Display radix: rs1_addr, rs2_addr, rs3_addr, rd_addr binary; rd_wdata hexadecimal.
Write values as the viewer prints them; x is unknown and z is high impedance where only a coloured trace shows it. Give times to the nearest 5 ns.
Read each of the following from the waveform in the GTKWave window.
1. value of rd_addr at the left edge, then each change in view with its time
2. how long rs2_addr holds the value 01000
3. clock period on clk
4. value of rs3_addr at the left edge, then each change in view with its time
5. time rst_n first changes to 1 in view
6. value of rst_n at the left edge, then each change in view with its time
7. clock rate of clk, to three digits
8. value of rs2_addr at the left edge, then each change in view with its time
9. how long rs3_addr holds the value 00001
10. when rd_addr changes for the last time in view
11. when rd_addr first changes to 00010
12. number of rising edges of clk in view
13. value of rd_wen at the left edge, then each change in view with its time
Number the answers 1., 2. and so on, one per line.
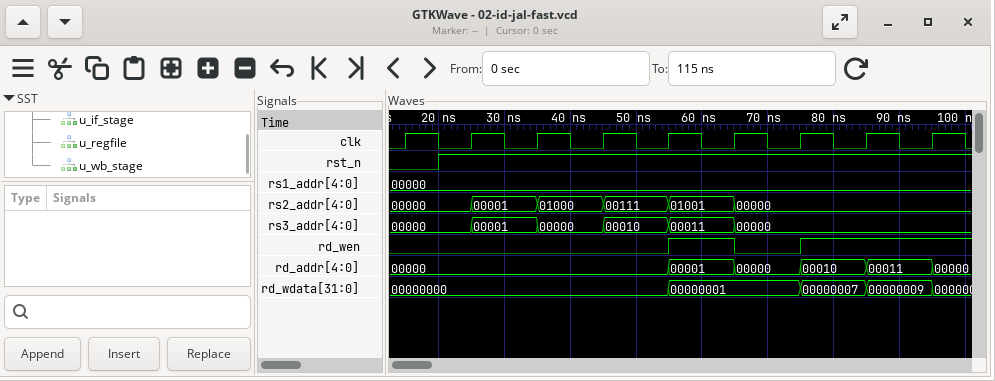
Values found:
1. 00000, 00001 at 55 ns, 00000 at 65 ns, 00010 at 75 ns, 00011 at 85 ns, 00000 at 95 ns
2. 10 ns
3. 10 ns
4. 00000, 00001 at 25 ns, 00000 at 35 ns, 00010 at 45 ns, 00011 at 55 ns, 00000 at 65 ns
5. 20 ns
6. 0, 1 at 20 ns
7. 100 MHz
8. 00000, 00001 at 25 ns, 01000 at 35 ns, 00111 at 45 ns, 01001 at 55 ns, 00000 at 65 ns
9. 10 ns
10. 95 ns
11. 75 ns
12. 9
13. 0, 1 at 55 ns, 0 at 65 ns, 1 at 75 ns
